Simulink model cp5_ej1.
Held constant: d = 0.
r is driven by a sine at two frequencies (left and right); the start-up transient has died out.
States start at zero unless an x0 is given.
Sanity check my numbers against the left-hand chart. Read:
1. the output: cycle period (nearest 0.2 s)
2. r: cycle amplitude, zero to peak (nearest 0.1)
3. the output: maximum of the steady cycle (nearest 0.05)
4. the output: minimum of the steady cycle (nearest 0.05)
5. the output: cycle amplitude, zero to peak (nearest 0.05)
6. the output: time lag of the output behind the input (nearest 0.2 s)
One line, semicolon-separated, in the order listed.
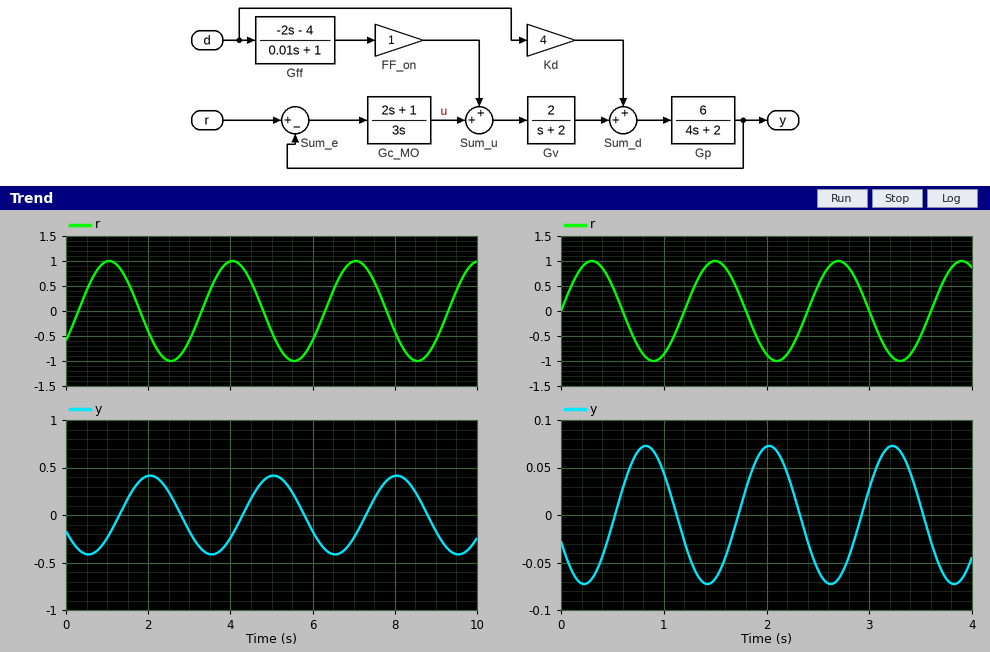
3.0 s; 1.0; 0.40; -0.40; 0.40; 1.0 s
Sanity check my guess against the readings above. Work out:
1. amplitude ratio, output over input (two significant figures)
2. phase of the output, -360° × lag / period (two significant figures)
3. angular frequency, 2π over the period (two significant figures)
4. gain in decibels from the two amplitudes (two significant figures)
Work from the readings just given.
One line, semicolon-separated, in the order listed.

0.40; -120°; 2.1 rad/s; -8.0 dB
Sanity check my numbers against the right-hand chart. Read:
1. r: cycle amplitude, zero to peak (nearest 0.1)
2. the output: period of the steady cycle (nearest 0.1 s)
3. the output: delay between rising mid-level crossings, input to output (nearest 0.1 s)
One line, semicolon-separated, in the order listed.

1.0; 1.2 s; 0.5 s
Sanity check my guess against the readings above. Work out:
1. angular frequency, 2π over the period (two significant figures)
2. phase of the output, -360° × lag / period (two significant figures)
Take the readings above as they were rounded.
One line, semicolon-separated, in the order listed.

5.2 rad/s; -150°
